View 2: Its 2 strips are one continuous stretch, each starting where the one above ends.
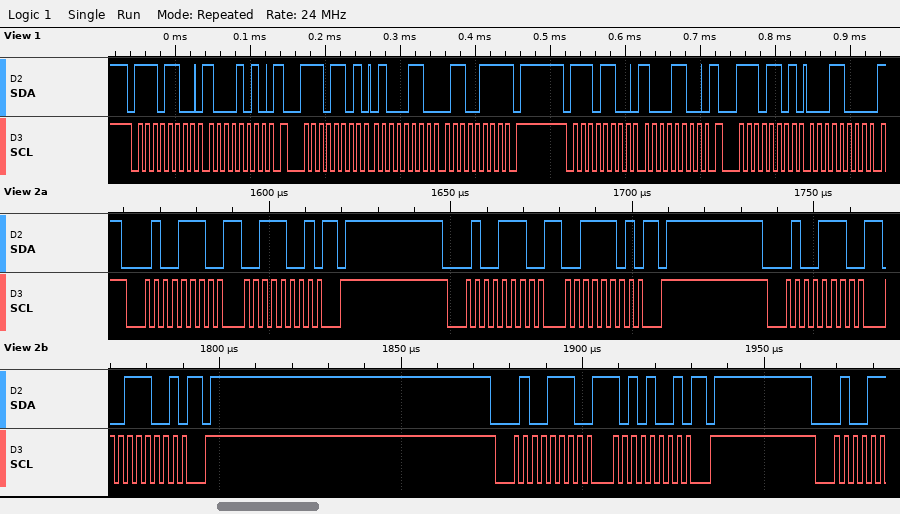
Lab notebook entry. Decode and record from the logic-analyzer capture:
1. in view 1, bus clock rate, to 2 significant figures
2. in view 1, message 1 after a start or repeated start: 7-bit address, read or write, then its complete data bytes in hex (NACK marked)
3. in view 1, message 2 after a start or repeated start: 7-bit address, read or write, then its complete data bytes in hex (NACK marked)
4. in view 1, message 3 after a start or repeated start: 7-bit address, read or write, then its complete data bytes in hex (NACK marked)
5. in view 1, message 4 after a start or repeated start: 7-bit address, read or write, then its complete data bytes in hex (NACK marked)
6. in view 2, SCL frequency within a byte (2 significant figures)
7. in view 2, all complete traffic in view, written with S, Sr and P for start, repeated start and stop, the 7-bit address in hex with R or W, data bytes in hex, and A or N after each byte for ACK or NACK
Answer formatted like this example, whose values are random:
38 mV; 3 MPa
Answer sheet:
100 kHz; 0x76 write: 8A; 0x76 read: 46 67 NACK; 0x76 write: 8C; 0x76 read: 18; 400 kHz; S 27W A 39 A P S 27W A 3D A P S 27W A 39 A P S 27W A A9 A P
